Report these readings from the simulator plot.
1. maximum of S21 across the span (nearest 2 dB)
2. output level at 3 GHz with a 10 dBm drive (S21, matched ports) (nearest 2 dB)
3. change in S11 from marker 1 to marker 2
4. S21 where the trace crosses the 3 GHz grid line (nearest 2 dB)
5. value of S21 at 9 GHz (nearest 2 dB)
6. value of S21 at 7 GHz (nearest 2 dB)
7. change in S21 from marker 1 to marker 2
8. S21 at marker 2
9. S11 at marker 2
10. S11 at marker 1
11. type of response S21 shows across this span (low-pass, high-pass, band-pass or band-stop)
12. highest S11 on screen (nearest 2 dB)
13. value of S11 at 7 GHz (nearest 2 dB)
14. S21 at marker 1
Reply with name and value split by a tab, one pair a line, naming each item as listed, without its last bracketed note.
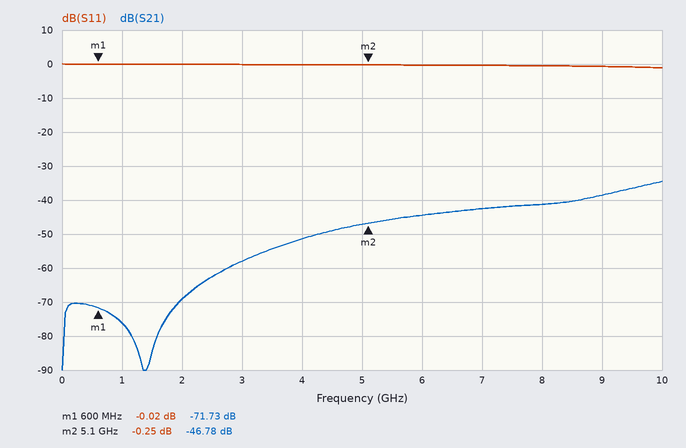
maximum of S21 across the span	-34 dB
output level at 3 GHz with a 10 dBm drive (S21, matched ports)	-48 dBm
change in S11 from marker 1 to marker 2	-0.23 dB
S21 where the trace crosses the 3 GHz grid line	-58 dB
value of S21 at 9 GHz	-38 dB
value of S21 at 7 GHz	-42 dB
change in S21 from marker 1 to marker 2	24.95 dB
S21 at marker 2	-46.78 dB
S11 at marker 2	-0.25 dB
S11 at marker 1	-0.02 dB
type of response S21 shows across this span	high-pass
highest S11 on screen	0 dB
value of S11 at 7 GHz	0 dB
S21 at marker 1	-71.73 dB
